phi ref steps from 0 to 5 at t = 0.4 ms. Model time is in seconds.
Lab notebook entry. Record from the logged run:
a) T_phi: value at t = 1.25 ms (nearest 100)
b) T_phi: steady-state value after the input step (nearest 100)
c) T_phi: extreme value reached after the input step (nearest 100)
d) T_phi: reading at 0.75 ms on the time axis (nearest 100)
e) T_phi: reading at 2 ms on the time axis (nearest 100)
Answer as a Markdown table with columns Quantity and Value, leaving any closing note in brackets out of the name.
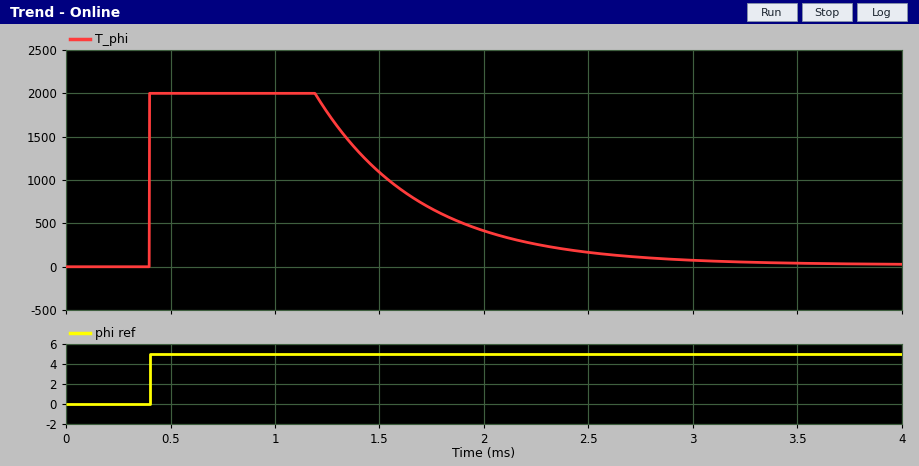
| Quantity | Value |
|---|---|
| T_phi: value at t = 1.25 ms | 1800 |
| T_phi: steady-state value after the input step | 0 |
| T_phi: extreme value reached after the input step | 2000 |
| T_phi: reading at 0.75 ms on the time axis | 2000 |
| T_phi: reading at 2 ms on the time axis | 400 |
